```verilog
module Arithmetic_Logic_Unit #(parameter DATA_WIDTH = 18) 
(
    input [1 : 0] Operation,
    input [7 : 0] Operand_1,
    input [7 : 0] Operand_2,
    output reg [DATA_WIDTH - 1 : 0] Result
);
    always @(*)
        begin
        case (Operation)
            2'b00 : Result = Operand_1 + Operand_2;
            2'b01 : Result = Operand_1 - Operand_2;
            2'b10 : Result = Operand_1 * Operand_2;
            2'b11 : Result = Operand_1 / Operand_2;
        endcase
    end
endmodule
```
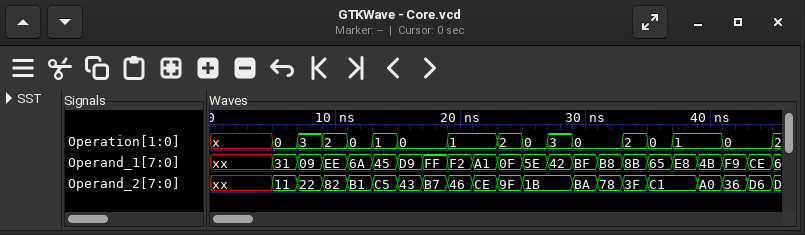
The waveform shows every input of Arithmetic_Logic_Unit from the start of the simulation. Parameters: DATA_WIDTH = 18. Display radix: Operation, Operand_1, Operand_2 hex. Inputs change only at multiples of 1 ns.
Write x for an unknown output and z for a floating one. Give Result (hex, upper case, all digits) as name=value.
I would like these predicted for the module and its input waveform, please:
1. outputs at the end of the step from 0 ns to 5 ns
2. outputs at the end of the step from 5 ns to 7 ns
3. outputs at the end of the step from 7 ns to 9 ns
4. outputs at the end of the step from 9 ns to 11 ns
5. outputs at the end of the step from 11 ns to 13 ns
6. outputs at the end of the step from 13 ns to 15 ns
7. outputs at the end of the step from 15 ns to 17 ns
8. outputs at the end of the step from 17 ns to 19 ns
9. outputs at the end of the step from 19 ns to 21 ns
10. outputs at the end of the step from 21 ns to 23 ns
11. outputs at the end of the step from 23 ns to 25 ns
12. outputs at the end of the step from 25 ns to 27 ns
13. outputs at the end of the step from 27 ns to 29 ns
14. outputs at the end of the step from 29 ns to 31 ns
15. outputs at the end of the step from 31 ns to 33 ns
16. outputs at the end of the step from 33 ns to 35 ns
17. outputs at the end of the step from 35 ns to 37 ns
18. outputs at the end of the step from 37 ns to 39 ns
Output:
Result=x
Result=00042
Result=00000
Result=078DC
Result=0011B
Result=3FF80
Result=0011C
Result=001B6
Result=000AC
Result=3FFD3
Result=00951
Result=00079
Result=00002
Result=00179
Result=00130
Result=02235
Result=00126
Result=00027
